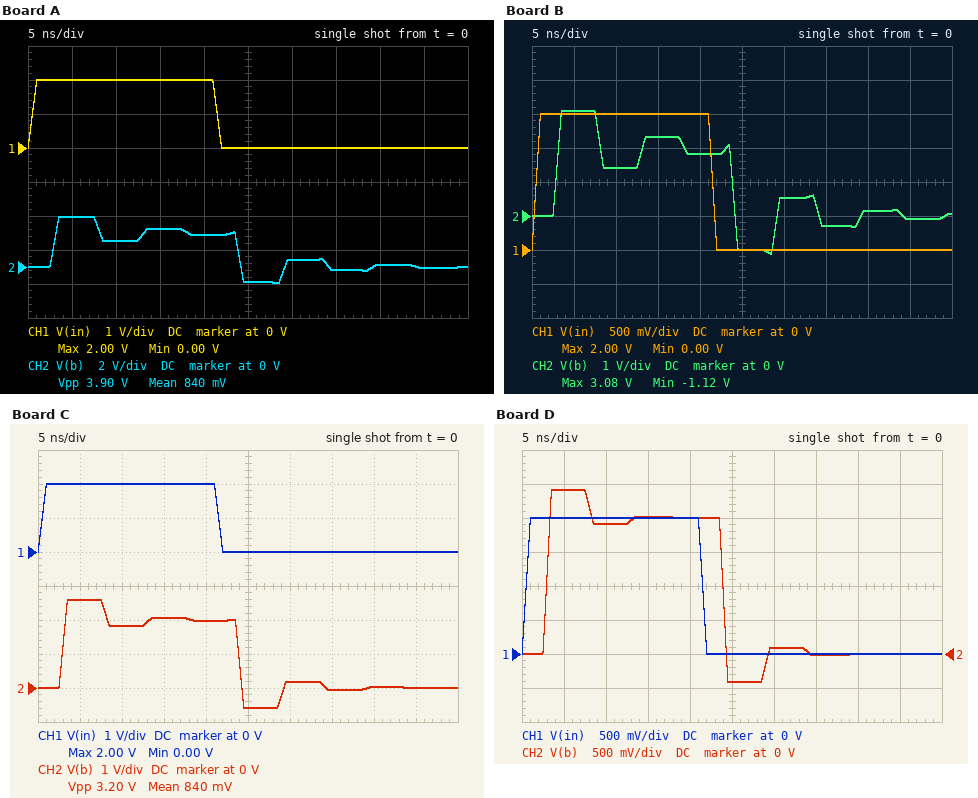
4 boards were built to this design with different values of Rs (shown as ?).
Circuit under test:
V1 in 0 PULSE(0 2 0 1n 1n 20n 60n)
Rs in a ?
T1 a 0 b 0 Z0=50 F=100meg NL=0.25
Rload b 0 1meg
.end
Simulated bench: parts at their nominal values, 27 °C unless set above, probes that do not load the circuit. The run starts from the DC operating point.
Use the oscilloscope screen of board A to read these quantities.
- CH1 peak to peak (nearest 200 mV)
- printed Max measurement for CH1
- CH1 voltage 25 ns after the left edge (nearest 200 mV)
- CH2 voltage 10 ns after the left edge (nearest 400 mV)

2.0 V
2.00 V
0 V
1.6 V
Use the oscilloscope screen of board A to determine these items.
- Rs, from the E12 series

18 Ω
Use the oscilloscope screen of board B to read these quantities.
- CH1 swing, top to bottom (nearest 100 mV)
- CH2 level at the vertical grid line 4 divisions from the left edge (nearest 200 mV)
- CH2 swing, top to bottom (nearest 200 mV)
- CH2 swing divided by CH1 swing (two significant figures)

2.0 V
1.8 V
4.2 V
2.1
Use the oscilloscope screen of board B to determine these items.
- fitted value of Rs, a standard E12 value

15 Ω
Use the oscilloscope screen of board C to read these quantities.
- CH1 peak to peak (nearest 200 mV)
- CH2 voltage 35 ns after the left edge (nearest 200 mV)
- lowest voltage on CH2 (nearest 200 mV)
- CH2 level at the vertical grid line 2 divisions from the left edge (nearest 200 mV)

2.0 V
0 V
-600 mV
1.8 V
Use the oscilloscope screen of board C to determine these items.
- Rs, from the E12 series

27 Ω
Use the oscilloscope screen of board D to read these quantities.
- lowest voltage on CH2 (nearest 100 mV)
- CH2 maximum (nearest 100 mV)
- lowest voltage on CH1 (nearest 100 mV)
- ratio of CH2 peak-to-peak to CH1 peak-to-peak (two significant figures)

-400 mV
2.4 V
0 V
1.4
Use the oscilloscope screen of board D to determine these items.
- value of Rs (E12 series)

33 Ω
